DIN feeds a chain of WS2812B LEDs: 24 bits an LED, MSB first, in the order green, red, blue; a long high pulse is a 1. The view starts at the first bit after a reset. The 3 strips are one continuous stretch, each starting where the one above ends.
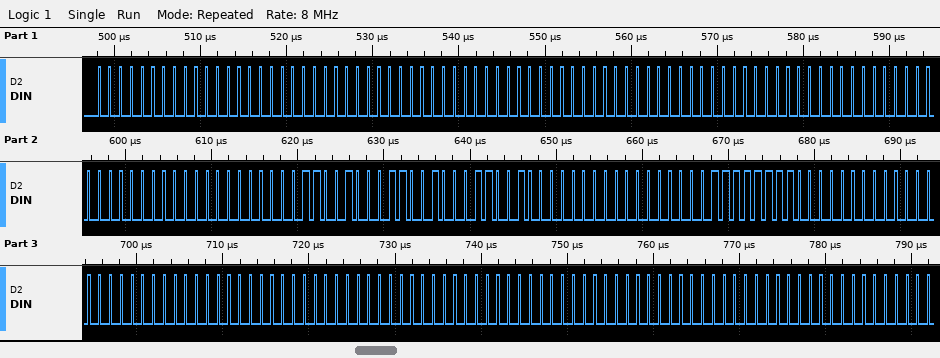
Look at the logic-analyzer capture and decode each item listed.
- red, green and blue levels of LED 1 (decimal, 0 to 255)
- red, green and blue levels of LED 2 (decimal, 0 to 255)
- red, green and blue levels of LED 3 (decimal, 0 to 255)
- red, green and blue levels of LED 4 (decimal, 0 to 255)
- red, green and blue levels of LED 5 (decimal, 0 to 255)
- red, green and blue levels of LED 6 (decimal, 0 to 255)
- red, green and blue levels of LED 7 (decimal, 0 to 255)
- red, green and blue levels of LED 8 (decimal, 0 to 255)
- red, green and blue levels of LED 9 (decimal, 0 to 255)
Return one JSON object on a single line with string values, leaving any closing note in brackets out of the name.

{"red, green and blue levels of LED 1": "0, 0, 0", "red, green and blue levels of LED 2": "0, 0, 0", "red, green and blue levels of LED 3": "0, 0, 0", "red, green and blue levels of LED 4": "0, 0, 0", "red, green and blue levels of LED 5": "50, 50, 50", "red, green and blue levels of LED 6": "0, 0, 255", "red, green and blue levels of LED 7": "0, 0, 0", "red, green and blue levels of LED 8": "0, 0, 0", "red, green and blue levels of LED 9": "0, 0, 0"}
